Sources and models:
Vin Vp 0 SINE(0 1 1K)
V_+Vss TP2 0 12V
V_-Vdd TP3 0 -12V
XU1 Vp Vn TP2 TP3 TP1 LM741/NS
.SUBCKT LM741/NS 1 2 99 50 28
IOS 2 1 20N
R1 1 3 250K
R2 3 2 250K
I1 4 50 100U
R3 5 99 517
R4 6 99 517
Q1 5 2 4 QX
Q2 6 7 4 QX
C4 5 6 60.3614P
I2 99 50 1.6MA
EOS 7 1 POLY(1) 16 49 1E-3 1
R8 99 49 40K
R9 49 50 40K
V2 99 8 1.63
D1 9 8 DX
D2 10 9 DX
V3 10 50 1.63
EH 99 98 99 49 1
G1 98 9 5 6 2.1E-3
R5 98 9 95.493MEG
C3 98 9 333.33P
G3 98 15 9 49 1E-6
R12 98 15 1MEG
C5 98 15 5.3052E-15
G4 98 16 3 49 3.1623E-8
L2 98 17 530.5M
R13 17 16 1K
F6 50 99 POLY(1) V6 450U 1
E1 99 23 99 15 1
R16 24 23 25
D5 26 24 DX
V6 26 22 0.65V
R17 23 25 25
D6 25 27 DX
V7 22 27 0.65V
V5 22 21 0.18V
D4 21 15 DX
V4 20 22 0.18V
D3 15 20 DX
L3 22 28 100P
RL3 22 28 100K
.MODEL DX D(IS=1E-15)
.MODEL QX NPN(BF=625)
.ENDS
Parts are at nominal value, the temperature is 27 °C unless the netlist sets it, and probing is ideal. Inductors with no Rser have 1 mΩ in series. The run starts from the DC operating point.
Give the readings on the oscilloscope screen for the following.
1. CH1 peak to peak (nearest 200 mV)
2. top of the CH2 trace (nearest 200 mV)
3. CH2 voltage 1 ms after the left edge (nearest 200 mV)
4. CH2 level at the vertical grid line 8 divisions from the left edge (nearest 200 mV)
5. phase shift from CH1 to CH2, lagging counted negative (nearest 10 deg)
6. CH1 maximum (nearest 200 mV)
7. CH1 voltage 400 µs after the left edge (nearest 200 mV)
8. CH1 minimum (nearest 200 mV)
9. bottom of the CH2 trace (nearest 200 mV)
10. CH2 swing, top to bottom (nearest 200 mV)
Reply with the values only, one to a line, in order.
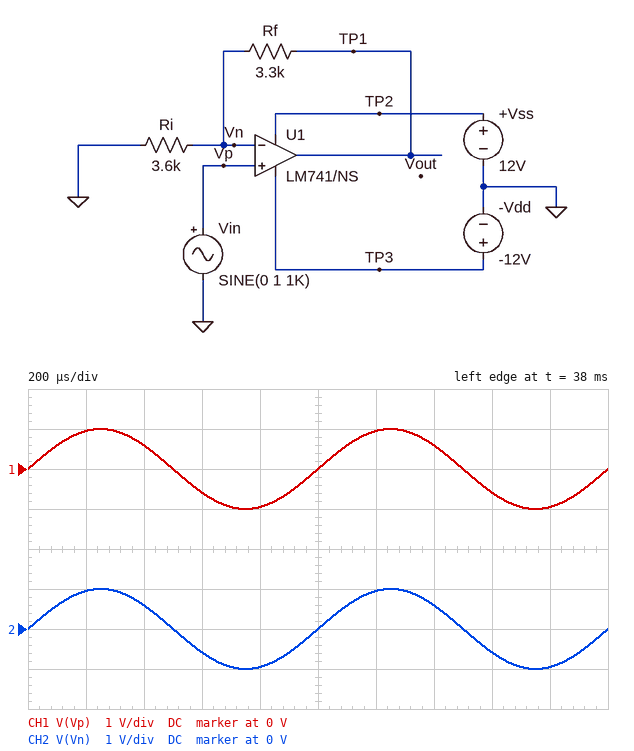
2.0 V
1.0 V
0 V
-600 mV
0 deg
1.0 V
600 mV
-1.0 V
-1.0 V
2.0 V
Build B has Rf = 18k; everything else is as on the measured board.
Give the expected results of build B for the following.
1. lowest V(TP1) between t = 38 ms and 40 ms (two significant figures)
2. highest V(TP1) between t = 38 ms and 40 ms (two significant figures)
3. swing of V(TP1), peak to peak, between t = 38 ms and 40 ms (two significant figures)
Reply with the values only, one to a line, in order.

-6.0 V
6.0 V
12 V
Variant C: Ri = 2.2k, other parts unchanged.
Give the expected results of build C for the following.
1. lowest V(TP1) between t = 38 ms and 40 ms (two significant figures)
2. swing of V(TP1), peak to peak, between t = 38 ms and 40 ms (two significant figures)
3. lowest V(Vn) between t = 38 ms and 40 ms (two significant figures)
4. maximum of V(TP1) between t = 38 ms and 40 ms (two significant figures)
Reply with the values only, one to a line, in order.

-2.5 V
5.0 V
-1.0 V
2.5 V
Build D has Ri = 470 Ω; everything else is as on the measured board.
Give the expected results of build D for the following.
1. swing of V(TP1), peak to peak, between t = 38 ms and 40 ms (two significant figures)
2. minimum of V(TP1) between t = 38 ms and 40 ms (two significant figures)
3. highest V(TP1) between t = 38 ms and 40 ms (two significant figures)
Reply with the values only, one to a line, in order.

16 V
-8.0 V
8.0 V
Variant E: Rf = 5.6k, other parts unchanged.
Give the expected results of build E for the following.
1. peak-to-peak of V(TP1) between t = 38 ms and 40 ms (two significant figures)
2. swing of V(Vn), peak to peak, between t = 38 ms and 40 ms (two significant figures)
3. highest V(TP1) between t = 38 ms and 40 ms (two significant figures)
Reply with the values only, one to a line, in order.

5.1 V
2.0 V
2.6 V
